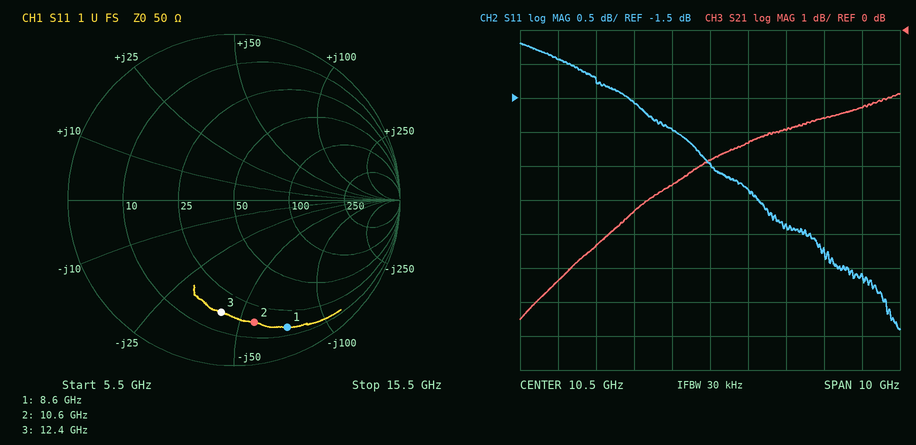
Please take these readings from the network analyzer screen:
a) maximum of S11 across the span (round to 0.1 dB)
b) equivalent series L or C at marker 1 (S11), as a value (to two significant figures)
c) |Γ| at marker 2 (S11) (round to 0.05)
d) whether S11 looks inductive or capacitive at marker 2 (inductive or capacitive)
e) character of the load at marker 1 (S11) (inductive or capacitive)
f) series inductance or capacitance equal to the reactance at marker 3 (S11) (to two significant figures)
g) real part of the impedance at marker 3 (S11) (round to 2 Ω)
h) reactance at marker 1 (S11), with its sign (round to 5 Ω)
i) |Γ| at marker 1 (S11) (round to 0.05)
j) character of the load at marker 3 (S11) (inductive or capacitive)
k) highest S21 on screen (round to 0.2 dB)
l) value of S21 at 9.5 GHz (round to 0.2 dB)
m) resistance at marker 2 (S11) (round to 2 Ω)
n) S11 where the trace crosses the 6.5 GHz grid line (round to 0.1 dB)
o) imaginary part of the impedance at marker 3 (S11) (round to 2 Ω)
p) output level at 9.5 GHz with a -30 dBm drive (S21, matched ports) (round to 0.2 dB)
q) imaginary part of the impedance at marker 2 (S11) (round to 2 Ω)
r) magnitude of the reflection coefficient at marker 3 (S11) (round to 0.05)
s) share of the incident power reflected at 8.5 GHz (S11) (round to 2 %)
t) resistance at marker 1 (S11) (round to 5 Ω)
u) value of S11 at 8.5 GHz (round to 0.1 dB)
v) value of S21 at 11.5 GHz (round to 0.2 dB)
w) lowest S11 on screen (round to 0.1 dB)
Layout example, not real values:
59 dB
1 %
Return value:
-0.7 dB
250 fF
0.75
capacitive
capacitive
310 fF
16 Ω
-75 Ω
0.85
capacitive
-1.8 dB
-4.6 dB
16 Ω
-0.9 dB
-42 Ω
-34.6 dBm
-56 Ω
0.70
70 %
15 Ω
-1.6 dB
-3.4 dB
-4.9 dB
